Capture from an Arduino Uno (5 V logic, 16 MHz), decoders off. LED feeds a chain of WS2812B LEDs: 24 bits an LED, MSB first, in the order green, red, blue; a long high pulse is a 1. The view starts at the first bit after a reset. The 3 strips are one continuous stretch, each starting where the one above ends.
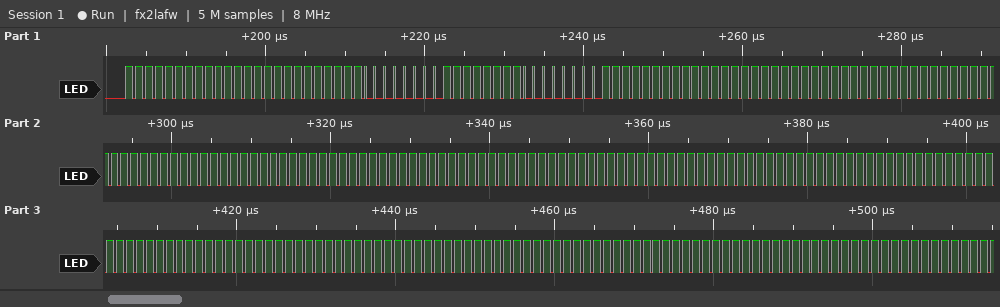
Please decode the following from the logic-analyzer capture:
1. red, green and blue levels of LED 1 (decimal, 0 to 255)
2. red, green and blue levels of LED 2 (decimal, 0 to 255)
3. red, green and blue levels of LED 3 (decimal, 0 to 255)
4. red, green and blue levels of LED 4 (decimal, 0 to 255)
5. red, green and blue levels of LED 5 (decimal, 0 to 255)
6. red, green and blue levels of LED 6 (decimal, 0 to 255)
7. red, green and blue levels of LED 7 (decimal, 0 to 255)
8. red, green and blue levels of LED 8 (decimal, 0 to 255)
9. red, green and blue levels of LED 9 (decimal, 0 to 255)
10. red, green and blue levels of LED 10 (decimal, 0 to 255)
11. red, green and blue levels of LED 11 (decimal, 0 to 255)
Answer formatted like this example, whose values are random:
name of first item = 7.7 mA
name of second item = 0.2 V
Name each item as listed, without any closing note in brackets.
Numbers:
red, green and blue levels of LED 1 = 255, 255, 255
red, green and blue levels of LED 2 = 255, 0, 0
red, green and blue levels of LED 3 = 255, 255, 255
red, green and blue levels of LED 4 = 255, 255, 255
red, green and blue levels of LED 5 = 255, 255, 255
red, green and blue levels of LED 6 = 255, 255, 255
red, green and blue levels of LED 7 = 255, 255, 255
red, green and blue levels of LED 8 = 255, 255, 255
red, green and blue levels of LED 9 = 255, 255, 255
red, green and blue levels of LED 10 = 255, 255, 255
red, green and blue levels of LED 11 = 255, 255, 255
